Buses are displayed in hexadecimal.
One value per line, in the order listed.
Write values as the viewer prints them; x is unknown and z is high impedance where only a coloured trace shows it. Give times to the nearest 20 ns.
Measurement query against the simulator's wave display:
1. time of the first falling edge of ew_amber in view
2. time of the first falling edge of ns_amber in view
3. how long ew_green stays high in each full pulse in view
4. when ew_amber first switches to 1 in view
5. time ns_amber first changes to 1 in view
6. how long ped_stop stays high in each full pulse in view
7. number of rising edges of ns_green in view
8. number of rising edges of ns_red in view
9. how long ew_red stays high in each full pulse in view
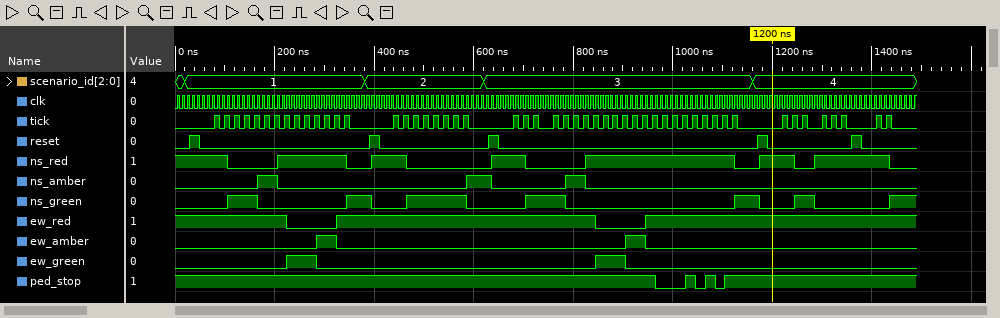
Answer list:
320 ns
200 ns
60 ns, 60 ns
280 ns
160 ns
20 ns, 20 ns
7
6
520 ns
